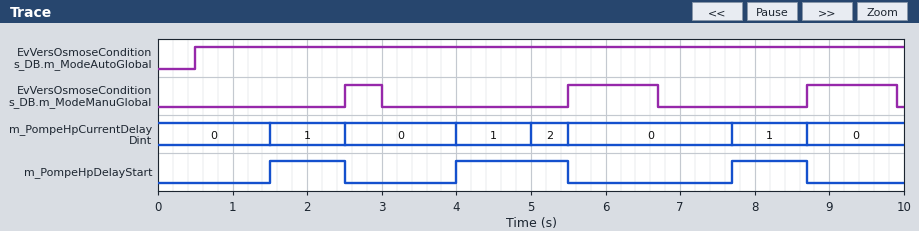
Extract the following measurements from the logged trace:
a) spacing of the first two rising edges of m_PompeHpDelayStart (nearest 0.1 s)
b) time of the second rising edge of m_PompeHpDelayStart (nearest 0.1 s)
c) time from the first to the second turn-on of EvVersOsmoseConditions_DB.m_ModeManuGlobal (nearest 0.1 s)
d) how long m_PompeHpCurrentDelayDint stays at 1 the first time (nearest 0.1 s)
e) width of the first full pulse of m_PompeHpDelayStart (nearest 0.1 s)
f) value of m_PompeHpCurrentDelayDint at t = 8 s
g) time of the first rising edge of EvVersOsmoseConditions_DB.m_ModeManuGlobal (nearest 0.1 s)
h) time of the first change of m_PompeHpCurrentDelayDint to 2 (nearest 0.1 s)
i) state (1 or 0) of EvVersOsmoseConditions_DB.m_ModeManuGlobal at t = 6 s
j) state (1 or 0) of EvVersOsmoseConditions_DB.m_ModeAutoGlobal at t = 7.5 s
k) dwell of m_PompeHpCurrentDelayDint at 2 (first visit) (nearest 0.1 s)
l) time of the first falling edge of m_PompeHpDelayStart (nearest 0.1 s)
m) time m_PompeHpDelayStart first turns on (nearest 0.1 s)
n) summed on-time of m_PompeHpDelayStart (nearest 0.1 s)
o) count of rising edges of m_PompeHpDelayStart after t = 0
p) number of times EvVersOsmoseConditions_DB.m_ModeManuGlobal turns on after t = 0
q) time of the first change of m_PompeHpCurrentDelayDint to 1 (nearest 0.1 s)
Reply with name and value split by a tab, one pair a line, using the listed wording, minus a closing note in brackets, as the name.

spacing of the first two rising edges of m_PompeHpDelayStart	2.5 s
time of the second rising edge of m_PompeHpDelayStart	4.0 s
time from the first to the second turn-on of EvVersOsmoseConditions_DB.m_ModeManuGlobal	3.0 s
how long m_PompeHpCurrentDelayDint stays at 1 the first time	1.0 s
width of the first full pulse of m_PompeHpDelayStart	1.0 s
value of m_PompeHpCurrentDelayDint at t = 8 s	1
time of the first rising edge of EvVersOsmoseConditions_DB.m_ModeManuGlobal	2.5 s
time of the first change of m_PompeHpCurrentDelayDint to 2	5.0 s
state (1 or 0) of EvVersOsmoseConditions_DB.m_ModeManuGlobal at t = 6 s	1
state (1 or 0) of EvVersOsmoseConditions_DB.m_ModeAutoGlobal at t = 7.5 s	1
dwell of m_PompeHpCurrentDelayDint at 2 (first visit)	0.5 s
time of the first falling edge of m_PompeHpDelayStart	2.5 s
time m_PompeHpDelayStart first turns on	1.5 s
summed on-time of m_PompeHpDelayStart	3.5 s
count of rising edges of m_PompeHpDelayStart after t = 0	3
number of times EvVersOsmoseConditions_DB.m_ModeManuGlobal turns on after t = 0	3
time of the first change of m_PompeHpCurrentDelayDint to 1	1.5 s
